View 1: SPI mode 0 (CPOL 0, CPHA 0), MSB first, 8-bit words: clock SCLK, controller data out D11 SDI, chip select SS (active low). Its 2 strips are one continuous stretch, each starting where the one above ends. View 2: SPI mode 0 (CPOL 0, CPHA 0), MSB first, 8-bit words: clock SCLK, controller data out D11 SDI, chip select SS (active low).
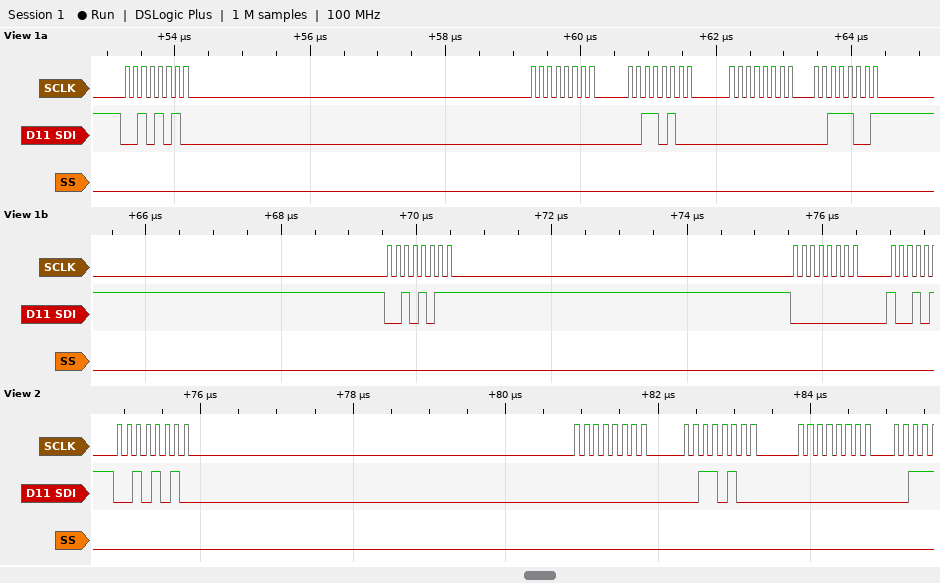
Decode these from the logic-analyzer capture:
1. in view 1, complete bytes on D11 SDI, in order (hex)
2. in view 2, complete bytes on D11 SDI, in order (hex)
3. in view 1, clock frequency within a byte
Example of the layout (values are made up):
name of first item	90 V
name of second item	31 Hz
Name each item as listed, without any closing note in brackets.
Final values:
in view 1, complete bytes on D11 SDI, in order	0x2A 0x00 0x34 0x00 0x39 0x2B 0x00
in view 2, complete bytes on D11 SDI, in order	2A 00 34 00
in view 1, clock frequency within a byte	8 MHz
